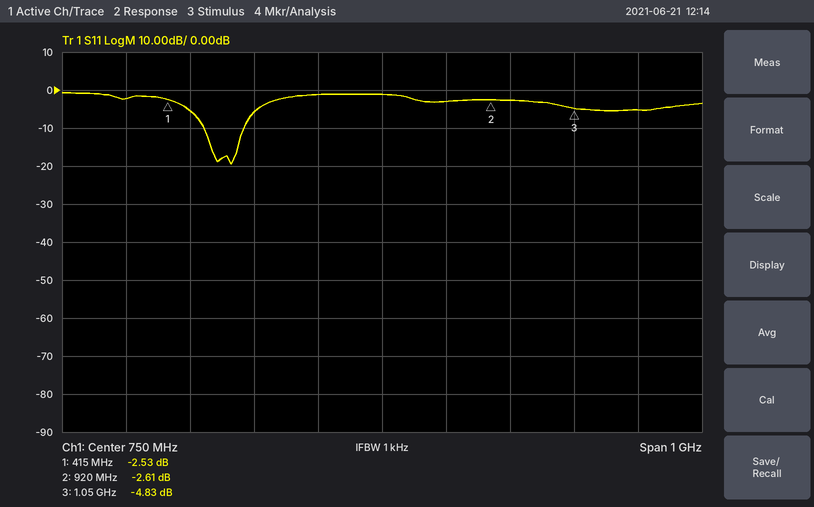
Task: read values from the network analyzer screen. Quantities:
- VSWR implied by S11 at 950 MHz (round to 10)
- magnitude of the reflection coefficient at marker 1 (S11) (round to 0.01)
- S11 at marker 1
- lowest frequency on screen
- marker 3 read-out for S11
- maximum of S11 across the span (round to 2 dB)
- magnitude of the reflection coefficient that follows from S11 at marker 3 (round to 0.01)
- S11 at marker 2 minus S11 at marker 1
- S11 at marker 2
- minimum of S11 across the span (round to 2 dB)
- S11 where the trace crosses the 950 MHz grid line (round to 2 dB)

10
0.75
-2.53 dB
250 MHz
-4.83 dB
0 dB
0.57
-0.08 dB
-2.61 dB
-20 dB
-2 dB
